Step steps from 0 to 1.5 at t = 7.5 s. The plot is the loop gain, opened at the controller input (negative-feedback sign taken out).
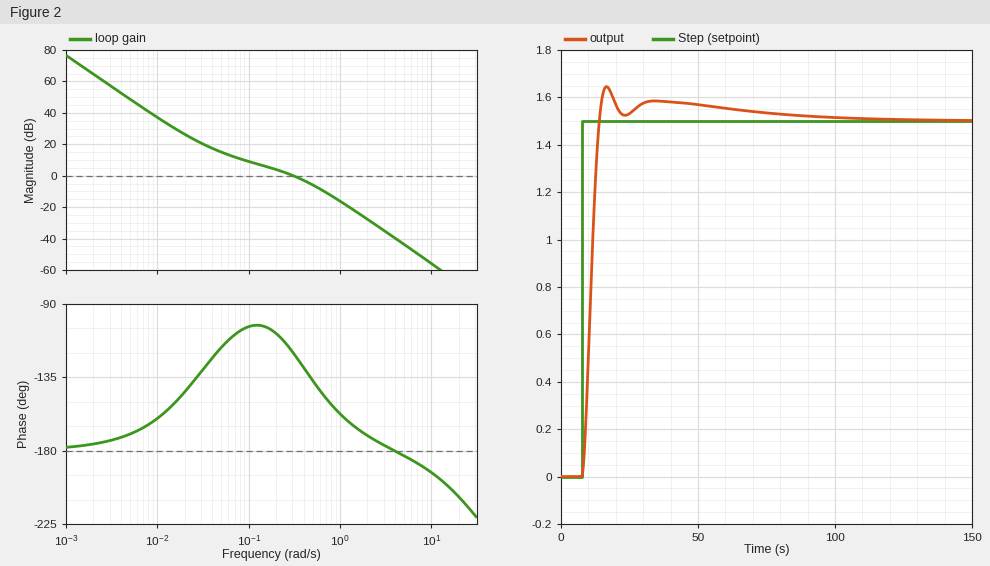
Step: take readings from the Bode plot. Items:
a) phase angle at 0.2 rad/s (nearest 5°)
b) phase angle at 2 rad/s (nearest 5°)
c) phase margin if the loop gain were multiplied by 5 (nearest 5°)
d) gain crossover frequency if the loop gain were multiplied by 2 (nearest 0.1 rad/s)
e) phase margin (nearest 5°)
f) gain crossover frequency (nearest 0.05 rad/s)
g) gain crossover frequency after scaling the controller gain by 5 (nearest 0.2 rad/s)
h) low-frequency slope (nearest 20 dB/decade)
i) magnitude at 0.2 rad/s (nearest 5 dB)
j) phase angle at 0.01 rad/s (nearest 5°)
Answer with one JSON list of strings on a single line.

["-110°", "-170°", "25°", "0.5 rad/s", "60°", "0.30 rad/s", "0.8 rad/s", "-40 dB/decade", "5 dB", "-160°"]
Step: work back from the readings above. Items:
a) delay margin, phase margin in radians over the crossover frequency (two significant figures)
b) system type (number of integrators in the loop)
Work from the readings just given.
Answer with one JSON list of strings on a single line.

["3.5 s", "2"]
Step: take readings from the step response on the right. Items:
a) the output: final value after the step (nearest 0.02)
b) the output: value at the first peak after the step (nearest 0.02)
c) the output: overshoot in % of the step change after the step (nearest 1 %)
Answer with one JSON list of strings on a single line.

["1.50", "1.64", "10 %"]
